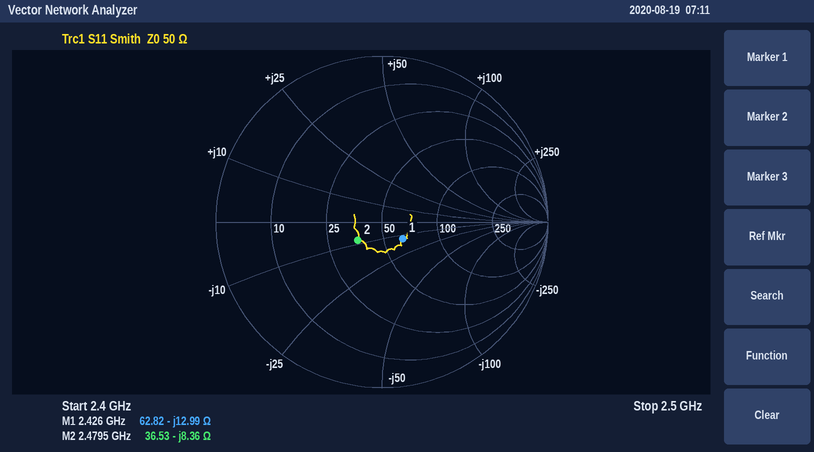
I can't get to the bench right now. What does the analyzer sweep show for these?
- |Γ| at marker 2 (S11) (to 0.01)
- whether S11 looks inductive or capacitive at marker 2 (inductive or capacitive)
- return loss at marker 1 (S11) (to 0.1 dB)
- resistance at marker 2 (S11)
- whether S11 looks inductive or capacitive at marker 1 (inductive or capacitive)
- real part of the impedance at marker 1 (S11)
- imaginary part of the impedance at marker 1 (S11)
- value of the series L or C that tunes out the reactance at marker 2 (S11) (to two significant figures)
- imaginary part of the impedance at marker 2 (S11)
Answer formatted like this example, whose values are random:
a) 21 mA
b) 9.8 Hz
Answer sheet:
a) 0.18
b) capacitive
c) 15.9 dB
d) 36.53 Ω
e) capacitive
f) 62.82 Ω
g) -12.99 Ω
h) 540 pH
i) -8.36 Ω
